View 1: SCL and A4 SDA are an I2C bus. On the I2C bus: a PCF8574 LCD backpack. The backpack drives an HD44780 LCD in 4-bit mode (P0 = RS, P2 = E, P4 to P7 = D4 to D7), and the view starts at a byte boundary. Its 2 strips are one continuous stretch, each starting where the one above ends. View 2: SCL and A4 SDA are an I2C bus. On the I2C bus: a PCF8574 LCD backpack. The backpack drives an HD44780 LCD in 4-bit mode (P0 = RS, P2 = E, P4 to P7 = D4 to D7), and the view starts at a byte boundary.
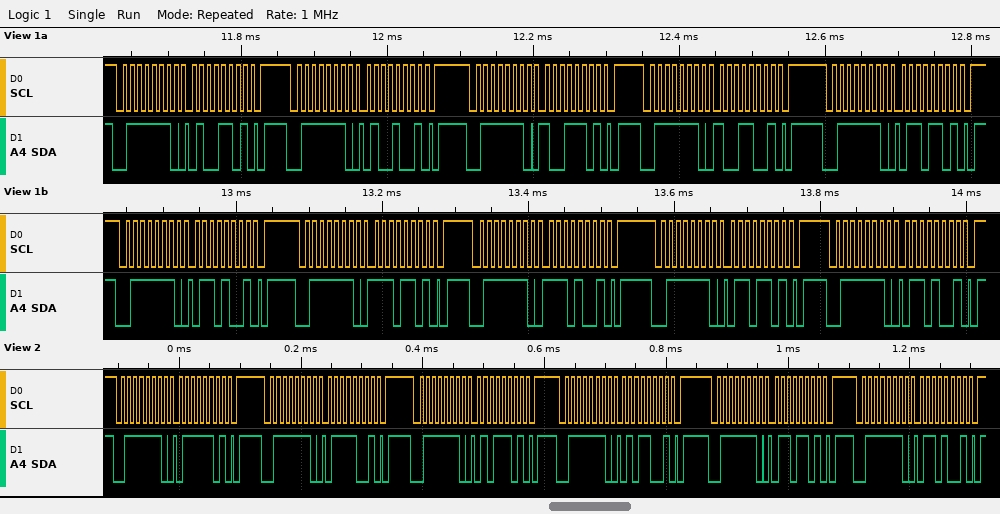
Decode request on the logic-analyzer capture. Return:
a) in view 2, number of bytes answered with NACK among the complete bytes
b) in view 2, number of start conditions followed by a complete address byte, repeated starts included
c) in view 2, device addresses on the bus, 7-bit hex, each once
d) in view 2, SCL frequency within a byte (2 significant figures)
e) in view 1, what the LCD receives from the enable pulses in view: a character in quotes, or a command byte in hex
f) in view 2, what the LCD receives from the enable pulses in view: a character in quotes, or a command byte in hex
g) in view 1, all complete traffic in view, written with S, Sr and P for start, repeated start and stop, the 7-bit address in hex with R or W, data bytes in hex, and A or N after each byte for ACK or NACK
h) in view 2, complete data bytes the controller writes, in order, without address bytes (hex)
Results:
0
6
0x3F
100 kHz
'I' 'n'
'u'
S 3FW A 4D A P S 3FW A 49 A P S 3FW A 9D A P S 3FW A 99 A P S 3FW A 6D A P S 3FW A 69 A P S 3FW A ED A P S 3FW A E9 A P S 3FW A 6D A P S 3FW A 69 A P
7D 79 5D 59 6D 69
